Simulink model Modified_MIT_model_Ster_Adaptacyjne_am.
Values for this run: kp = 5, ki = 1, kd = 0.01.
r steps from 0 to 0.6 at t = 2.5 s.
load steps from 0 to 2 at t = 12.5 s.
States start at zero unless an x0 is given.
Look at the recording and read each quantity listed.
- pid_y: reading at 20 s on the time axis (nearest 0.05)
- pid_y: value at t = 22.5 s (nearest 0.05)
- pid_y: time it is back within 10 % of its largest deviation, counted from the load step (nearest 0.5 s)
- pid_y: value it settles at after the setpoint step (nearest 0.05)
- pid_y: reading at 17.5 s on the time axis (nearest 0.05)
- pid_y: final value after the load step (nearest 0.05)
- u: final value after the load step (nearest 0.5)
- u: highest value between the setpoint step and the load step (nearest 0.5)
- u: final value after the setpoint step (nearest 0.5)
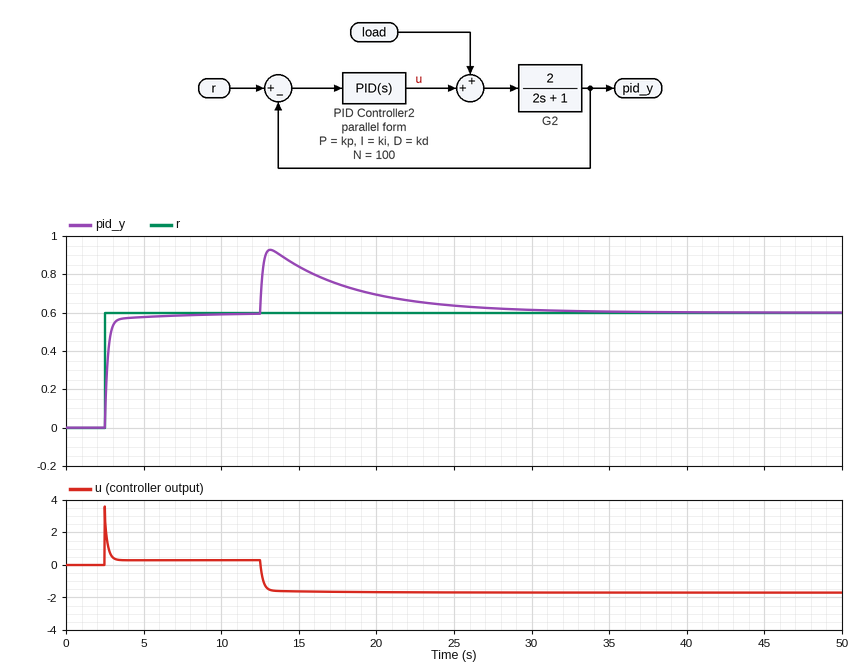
0.70
0.65
13.0 s
0.60
0.75
0.60
-1.5
3.5
0.5
